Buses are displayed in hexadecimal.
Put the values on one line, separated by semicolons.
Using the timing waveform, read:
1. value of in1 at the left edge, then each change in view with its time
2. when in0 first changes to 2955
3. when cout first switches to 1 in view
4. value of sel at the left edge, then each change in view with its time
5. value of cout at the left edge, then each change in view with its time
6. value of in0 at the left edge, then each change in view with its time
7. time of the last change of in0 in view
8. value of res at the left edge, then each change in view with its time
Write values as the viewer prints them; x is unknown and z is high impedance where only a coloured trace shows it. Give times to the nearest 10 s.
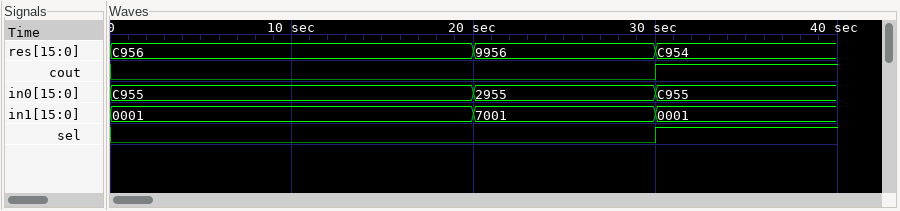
0001, 7001 at 20 s, 0001 at 30 s; 20 s; 30 s; 0, 1 at 30 s; 0, 1 at 30 s; C955, 2955 at 20 s, C955 at 30 s; 30 s; C956, 9956 at 20 s, C954 at 30 s
